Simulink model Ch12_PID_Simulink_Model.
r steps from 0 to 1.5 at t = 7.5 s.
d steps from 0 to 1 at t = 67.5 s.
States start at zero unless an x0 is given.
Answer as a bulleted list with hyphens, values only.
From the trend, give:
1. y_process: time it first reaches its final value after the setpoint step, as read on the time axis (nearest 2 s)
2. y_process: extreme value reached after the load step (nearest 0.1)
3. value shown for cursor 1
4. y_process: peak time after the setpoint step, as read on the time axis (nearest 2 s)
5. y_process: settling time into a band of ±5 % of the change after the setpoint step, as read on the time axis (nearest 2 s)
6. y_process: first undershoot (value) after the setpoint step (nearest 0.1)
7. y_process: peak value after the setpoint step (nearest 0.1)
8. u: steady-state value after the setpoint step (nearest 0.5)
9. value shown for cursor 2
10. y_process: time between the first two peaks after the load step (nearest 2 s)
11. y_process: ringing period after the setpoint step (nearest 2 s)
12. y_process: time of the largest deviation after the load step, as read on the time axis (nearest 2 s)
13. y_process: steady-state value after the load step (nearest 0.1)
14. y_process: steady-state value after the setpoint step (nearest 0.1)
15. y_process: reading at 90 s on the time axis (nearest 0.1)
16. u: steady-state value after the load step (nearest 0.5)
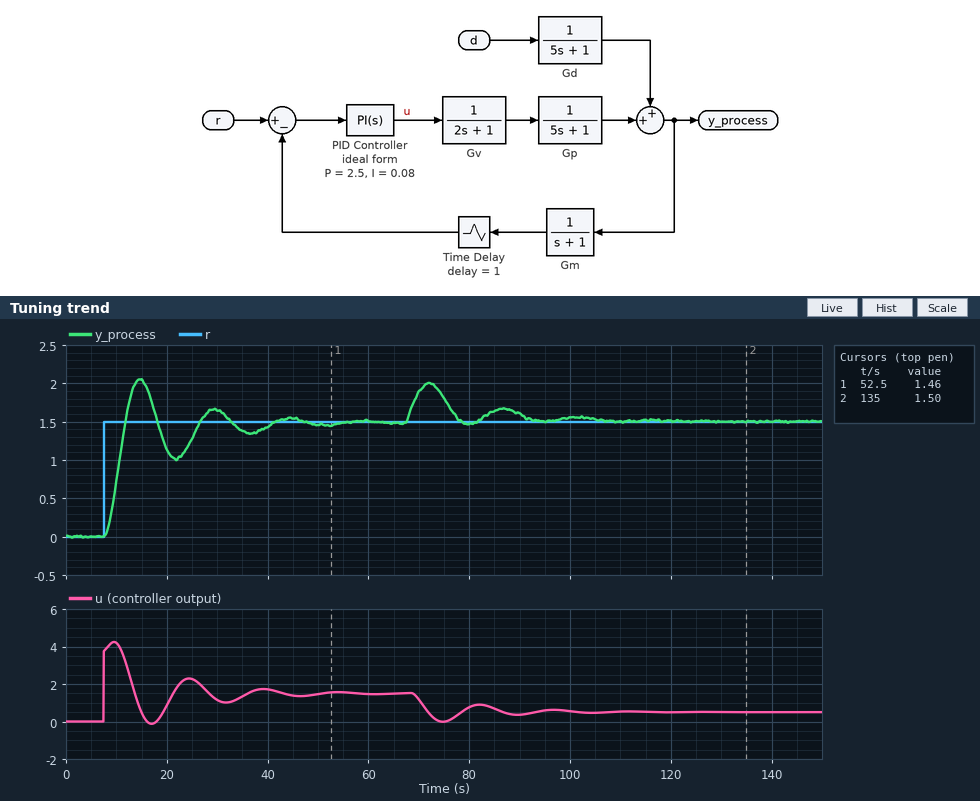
- 12 s
- 2.0
- 1.46
- 14 s
- 40 s
- 1.0
- 2.1
- 1.5
- 1.50
- 14 s
- 14 s
- 72 s
- 1.5
- 1.5
- 1.6
- 0.5
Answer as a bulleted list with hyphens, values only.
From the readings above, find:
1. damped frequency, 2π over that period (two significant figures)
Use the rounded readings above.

- 0.45 rad/s
